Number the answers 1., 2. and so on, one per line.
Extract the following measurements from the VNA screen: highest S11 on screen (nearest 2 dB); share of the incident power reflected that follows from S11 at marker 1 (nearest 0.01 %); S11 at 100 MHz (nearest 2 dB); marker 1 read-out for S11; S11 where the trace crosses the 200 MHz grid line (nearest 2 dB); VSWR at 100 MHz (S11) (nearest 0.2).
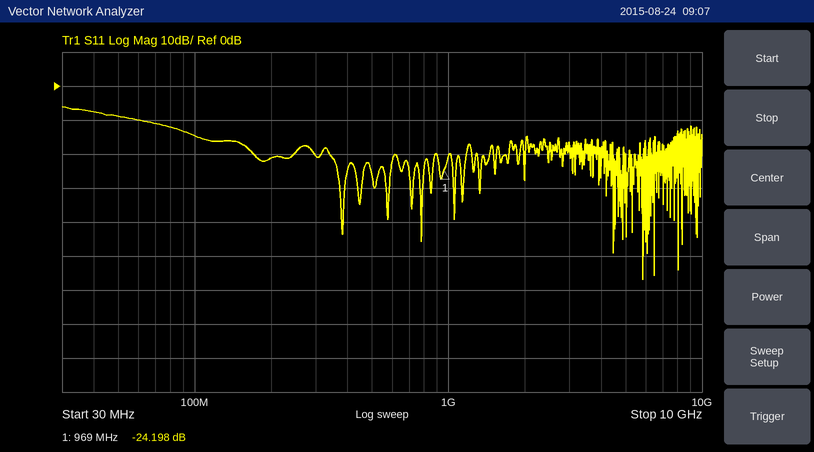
1. -6 dB
2. 0.38 %
3. -14 dB
4. -24.198 dB
5. -22 dB
6. 1.4
